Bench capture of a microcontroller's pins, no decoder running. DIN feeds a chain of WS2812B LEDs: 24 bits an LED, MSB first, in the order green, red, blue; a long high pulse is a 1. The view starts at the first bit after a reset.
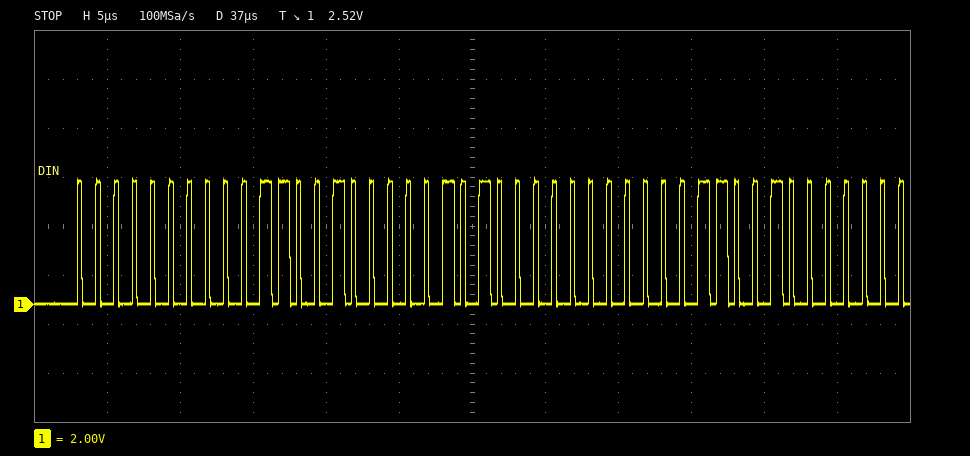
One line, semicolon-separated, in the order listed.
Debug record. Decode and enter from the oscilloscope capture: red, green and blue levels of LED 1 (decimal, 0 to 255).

50, 0, 10
